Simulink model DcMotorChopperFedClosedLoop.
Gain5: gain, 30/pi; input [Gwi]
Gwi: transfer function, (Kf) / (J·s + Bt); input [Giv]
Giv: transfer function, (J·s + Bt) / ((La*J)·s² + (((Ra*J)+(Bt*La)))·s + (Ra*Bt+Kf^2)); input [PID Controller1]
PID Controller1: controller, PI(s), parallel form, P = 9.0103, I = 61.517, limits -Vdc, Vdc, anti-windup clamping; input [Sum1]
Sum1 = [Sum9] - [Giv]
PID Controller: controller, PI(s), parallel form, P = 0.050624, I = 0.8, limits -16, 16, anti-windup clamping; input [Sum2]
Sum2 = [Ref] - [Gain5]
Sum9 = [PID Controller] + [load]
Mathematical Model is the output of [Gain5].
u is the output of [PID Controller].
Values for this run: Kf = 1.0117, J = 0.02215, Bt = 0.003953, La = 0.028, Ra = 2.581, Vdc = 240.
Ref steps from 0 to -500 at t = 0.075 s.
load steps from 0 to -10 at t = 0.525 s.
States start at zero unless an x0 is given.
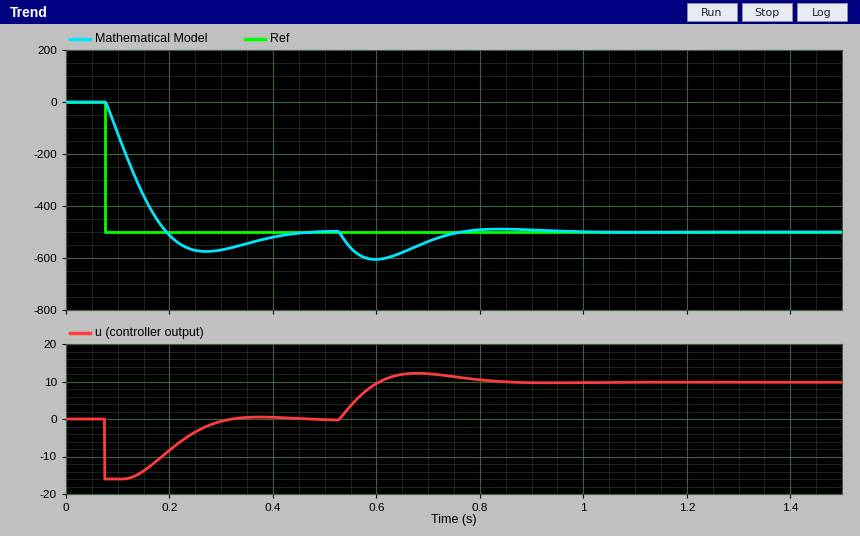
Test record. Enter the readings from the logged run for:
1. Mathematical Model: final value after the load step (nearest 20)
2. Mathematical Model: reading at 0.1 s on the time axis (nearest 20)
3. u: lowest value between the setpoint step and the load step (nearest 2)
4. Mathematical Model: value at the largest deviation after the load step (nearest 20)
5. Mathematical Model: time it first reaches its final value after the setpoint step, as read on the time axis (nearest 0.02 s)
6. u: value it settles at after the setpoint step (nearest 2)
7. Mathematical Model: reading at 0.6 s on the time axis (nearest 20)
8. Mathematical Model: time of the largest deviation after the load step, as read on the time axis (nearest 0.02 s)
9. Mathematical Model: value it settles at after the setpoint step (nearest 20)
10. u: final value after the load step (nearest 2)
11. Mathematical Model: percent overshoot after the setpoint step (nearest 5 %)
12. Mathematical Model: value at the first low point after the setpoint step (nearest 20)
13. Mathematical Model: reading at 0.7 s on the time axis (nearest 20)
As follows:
-500
-120
-16
-600
0.20 s
0
-600
0.60 s
-500
10
15 %
-580
-540
